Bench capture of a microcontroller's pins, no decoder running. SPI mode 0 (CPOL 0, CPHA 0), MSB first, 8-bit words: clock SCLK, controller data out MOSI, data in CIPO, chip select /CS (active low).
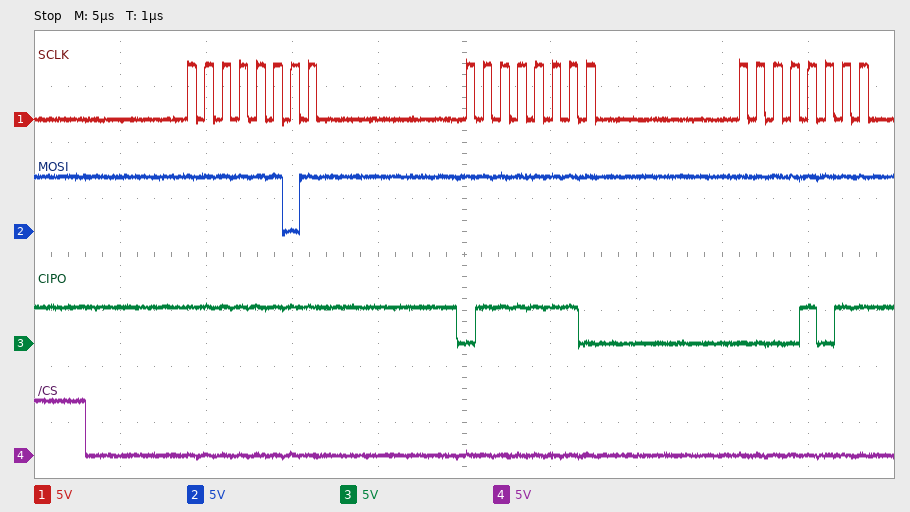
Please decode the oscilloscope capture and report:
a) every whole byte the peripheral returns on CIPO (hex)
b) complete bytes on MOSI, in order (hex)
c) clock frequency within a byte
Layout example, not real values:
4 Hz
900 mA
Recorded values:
FF 7E 0B
FD FF FF
1 MHz
